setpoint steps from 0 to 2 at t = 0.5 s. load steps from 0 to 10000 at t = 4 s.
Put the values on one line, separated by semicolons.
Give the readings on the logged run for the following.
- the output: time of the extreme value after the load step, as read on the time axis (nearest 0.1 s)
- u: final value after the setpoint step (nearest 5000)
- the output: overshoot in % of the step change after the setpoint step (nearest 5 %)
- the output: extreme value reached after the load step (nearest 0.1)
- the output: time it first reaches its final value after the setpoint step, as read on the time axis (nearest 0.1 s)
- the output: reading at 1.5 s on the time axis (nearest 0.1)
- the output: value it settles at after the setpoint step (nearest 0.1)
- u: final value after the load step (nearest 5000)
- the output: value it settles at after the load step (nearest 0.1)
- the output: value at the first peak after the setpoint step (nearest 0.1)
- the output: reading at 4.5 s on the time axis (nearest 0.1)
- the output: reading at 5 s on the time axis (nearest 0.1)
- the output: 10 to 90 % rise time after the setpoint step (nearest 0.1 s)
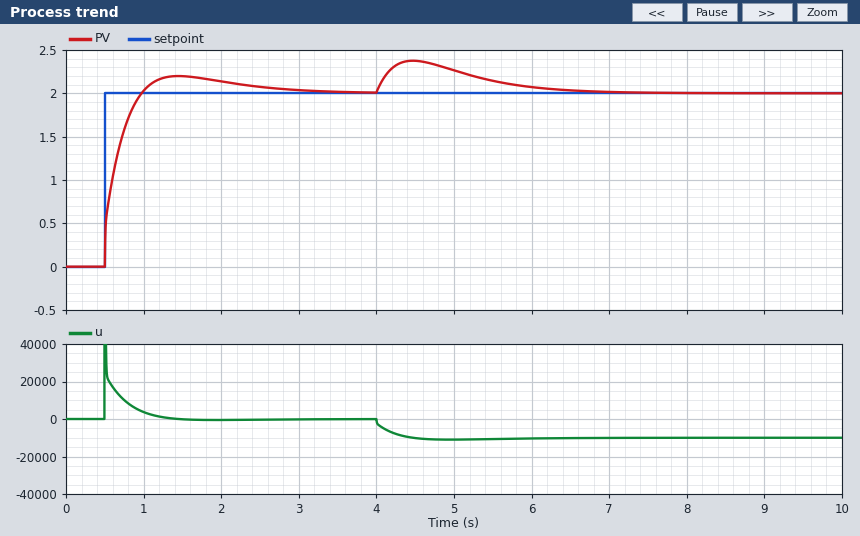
4.5 s; 0; 10 %; 2.4; 1.0 s; 2.2; 2.0; -10000; 2.0; 2.2; 2.4; 2.3; 0.3 s
